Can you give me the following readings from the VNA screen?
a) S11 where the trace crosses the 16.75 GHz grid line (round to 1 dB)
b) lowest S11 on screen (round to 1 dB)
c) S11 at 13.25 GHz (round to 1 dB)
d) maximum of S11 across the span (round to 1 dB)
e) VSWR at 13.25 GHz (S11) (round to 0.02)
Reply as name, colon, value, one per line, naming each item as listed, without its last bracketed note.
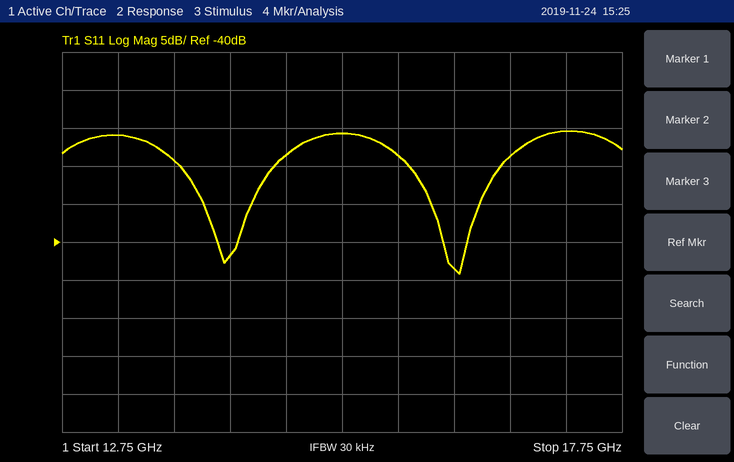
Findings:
S11 where the trace crosses the 16.75 GHz grid line: -29 dB
lowest S11 on screen: -44 dB
S11 at 13.25 GHz: -26 dB
maximum of S11 across the span: -25 dB
VSWR at 13.25 GHz (S11): 1.10
